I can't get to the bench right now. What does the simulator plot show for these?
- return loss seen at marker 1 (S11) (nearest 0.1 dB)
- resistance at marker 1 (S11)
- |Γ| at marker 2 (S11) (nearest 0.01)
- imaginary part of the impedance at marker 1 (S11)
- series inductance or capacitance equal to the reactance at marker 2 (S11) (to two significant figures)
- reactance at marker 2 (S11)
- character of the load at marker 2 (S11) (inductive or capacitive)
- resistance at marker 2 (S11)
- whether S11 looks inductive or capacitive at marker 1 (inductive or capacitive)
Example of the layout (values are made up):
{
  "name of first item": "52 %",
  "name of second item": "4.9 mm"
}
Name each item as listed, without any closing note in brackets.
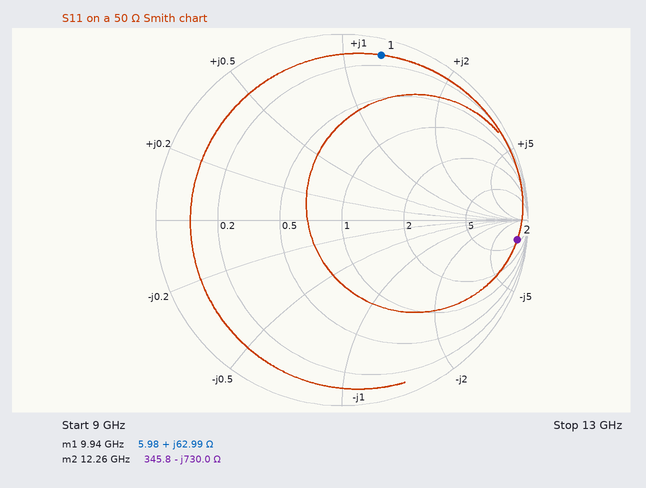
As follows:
{
  "return loss seen at marker 1 (S11)": "0.8 dB",
  "resistance at marker 1": "5.98 Ω",
  "|Γ| at marker 2 (S11)": "0.95",
  "imaginary part of the impedance at marker 1": "+62.99 Ω",
  "series inductance or capacitance equal to the reactance at marker 2 (S11)": "18 fF",
  "reactance at marker 2": "-730.0 Ω",
  "character of the load at marker 2 (S11)": "capacitive",
  "resistance at marker 2": "345.8 Ω",
  "whether S11 looks inductive or capacitive at marker 1": "inductive"
}
